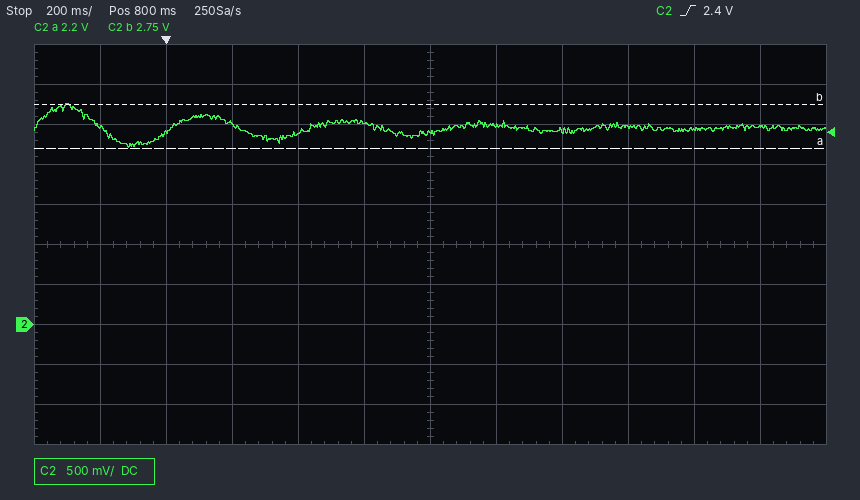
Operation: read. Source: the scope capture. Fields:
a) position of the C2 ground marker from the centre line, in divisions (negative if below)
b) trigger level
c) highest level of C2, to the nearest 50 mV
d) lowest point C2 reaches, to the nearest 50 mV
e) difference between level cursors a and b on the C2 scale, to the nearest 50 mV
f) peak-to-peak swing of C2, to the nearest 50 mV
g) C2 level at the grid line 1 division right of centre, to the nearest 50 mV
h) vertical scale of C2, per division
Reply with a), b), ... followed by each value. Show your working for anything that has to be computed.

a) -2.0 div
b) 2.4 V
c) 2.75 V
d) 2.20 V
e) 550 mV
f) 2.75 V − (2.20 V) = 550 mV
g) 2.50 V
h) 500 mV
